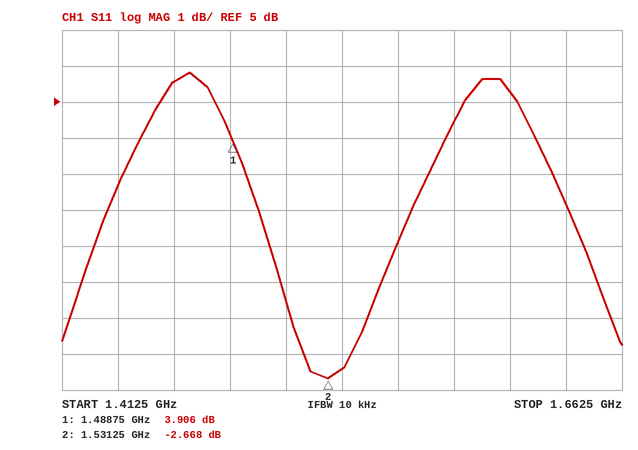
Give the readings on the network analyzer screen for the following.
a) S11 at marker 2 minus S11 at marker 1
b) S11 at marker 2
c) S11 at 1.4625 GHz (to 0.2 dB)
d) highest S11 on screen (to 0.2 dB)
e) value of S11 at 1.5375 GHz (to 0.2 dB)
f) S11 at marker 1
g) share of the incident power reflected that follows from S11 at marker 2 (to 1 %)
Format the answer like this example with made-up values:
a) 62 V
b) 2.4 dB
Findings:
a) -6.574 dB
b) -2.668 dB
c) 5.6 dB
d) 5.8 dB
e) -2.4 dB
f) 3.906 dB
g) 54 %
